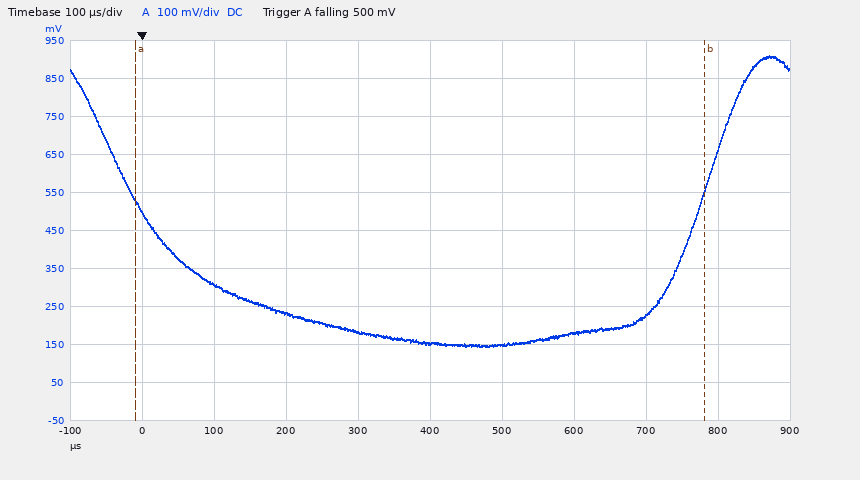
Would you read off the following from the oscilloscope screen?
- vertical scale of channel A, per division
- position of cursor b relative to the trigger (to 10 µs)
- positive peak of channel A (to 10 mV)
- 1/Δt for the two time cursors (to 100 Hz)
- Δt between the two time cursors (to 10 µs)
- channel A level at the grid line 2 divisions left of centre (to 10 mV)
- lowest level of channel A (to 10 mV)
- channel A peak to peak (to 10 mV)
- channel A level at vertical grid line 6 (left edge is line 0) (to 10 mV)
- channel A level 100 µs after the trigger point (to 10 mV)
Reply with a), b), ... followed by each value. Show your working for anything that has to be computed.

a) 100 mV
b) +780 µs
c) 910 mV
d) 1 / 790 µs ≈ 1.3 kHz
e) 790 µs
f) 230 mV
g) 140 mV
h) 910 mV − (140 mV) = 770 mV
i) 150 mV
j) 310 mV
